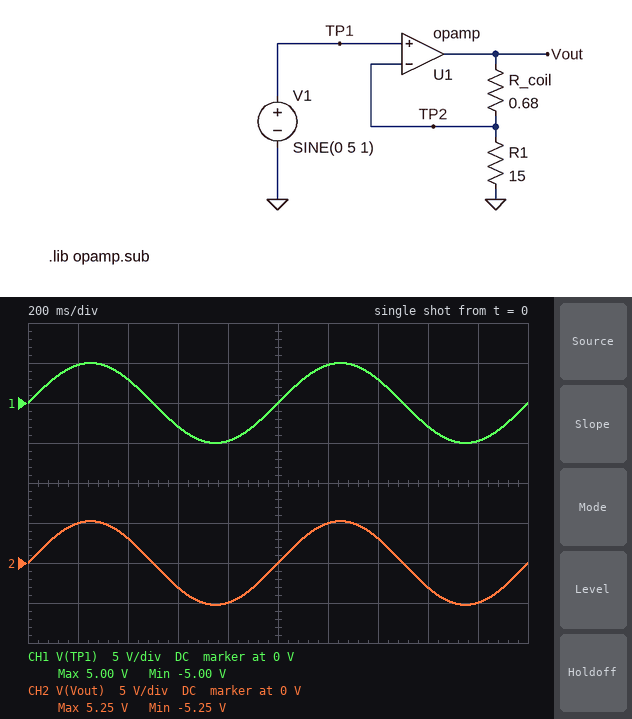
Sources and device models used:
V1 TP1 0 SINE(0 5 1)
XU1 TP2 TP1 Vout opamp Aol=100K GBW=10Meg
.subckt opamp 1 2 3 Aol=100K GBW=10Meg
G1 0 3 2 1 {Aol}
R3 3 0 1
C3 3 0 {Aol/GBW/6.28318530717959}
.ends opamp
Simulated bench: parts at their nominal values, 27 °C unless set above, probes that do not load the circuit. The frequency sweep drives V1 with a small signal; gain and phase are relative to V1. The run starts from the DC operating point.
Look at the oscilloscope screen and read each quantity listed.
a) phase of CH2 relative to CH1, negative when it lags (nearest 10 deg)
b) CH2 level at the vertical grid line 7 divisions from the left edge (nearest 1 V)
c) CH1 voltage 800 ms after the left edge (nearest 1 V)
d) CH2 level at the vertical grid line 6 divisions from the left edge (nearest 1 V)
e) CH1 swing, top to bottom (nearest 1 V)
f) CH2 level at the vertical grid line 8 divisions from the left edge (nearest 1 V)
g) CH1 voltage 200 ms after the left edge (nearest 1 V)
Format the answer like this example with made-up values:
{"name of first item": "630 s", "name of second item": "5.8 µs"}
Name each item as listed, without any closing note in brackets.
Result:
{"phase of CH2 relative to CH1, negative when it lags": "0 deg", "CH2 level at the vertical grid line 7 divisions from the left edge": "3 V", "CH1 voltage 800 ms after the left edge": "-5 V", "CH2 level at the vertical grid line 6 divisions from the left edge": "5 V", "CH1 swing, top to bottom": "10 V", "CH2 level at the vertical grid line 8 divisions from the left edge": "-3 V", "CH1 voltage 200 ms after the left edge": "5 V"}
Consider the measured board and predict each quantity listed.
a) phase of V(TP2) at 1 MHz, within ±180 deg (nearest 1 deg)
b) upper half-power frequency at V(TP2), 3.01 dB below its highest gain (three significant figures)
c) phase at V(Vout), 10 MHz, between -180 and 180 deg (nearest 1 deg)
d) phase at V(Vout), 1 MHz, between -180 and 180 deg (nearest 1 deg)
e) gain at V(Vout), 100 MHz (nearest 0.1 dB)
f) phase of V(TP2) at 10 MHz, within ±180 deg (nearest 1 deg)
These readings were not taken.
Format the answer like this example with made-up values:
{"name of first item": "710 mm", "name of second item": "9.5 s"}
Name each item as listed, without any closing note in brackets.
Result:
{"phase of V(TP2) at 1 MHz, within ±180 deg": "-6 deg", "upper half-power frequency at V(TP2), 3.01 dB below its highest gain": "9.57 MHz", "phase at V(Vout), 10 MHz, between -180 and 180 deg": "-46 deg", "phase at V(Vout), 1 MHz, between -180 and 180 deg": "-6 deg", "gain at V(Vout), 100 MHz": "-20.0 dB", "phase of V(TP2) at 10 MHz, within ±180 deg": "-46 deg"}
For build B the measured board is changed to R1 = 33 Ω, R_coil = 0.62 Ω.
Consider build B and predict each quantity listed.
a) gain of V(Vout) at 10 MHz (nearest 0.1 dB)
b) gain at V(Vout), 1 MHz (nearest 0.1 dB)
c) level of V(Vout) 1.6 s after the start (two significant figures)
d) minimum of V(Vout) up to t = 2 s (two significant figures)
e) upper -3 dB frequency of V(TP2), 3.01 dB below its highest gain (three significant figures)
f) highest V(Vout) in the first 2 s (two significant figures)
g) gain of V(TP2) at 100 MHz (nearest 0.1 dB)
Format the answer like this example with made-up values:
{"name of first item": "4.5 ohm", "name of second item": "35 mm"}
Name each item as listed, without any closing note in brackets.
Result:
{"gain of V(Vout) at 10 MHz": "-2.9 dB", "gain at V(Vout), 1 MHz": "0.1 dB", "level of V(Vout) 1.6 s after the start": "-3.0 V", "minimum of V(Vout) up to t = 2 s": "-5.1 V", "upper -3 dB frequency of V(TP2), 3.01 dB below its highest gain": "9.82 MHz", "highest V(Vout) in the first 2 s": "5.1 V", "gain of V(TP2) at 100 MHz": "-20.2 dB"}
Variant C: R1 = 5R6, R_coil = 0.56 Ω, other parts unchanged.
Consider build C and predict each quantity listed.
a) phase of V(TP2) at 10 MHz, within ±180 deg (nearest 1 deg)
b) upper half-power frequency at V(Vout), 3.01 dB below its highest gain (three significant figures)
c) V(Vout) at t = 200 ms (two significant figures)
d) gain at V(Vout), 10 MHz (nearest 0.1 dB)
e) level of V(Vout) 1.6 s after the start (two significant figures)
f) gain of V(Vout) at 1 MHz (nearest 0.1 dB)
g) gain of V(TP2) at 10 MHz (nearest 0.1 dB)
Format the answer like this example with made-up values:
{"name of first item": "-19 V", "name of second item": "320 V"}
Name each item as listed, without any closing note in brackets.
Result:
{"phase of V(TP2) at 10 MHz, within ±180 deg": "-48 deg", "upper half-power frequency at V(Vout), 3.01 dB below its highest gain": "9.09 MHz", "V(Vout) at t = 200 ms": "5.2 V", "gain at V(Vout), 10 MHz": "-2.6 dB", "level of V(Vout) 1.6 s after the start": "-3.2 V", "gain of V(Vout) at 1 MHz": "0.8 dB", "gain of V(TP2) at 10 MHz": "-3.4 dB"}
